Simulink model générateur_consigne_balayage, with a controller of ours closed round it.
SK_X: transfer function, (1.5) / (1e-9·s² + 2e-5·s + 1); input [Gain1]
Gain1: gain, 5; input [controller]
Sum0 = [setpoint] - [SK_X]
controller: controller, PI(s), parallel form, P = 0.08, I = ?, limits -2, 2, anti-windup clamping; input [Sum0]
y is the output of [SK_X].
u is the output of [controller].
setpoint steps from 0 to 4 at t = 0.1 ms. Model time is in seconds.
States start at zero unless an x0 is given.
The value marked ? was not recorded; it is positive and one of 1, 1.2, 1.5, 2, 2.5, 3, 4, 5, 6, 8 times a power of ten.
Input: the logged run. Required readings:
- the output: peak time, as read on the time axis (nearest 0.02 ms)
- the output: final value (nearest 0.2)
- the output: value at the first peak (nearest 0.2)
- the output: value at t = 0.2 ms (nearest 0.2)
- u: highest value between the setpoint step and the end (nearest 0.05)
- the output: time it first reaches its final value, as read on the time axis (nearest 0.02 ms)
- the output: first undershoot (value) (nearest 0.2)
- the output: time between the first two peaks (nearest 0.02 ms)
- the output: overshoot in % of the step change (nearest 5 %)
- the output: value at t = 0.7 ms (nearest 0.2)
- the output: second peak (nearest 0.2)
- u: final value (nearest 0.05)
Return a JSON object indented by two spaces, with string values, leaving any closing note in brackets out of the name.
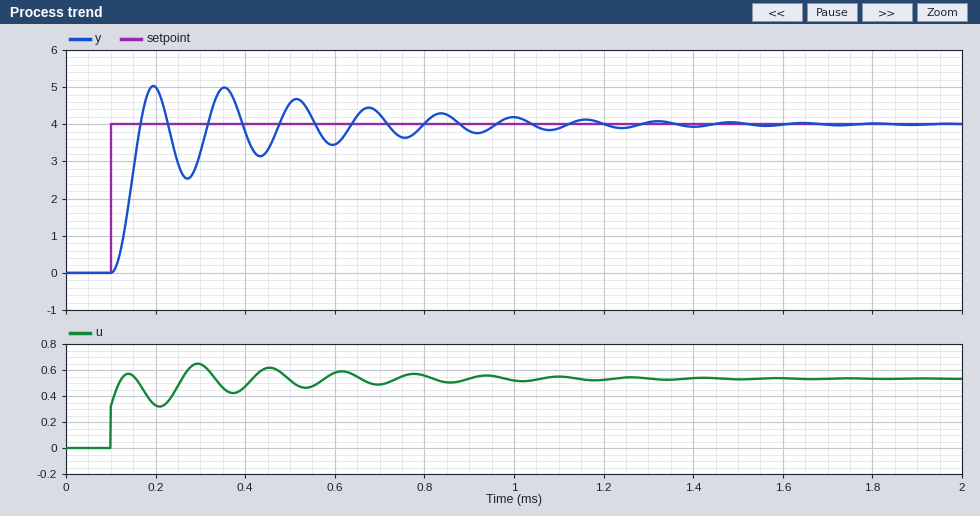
{
  "the output: peak time, as read on the time axis": "0.20 ms",
  "the output: final value": "4.0",
  "the output: value at the first peak": "5.0",
  "the output: value at t = 0.2 ms": "5.0",
  "u: highest value between the setpoint step and the end": "0.65",
  "the output: time it first reaches its final value, as read on the time axis": "0.16 ms",
  "the output: first undershoot (value)": "2.6",
  "the output: time between the first two peaks": "0.16 ms",
  "the output: overshoot in % of the step change": "25 %",
  "the output: value at t = 0.7 ms": "4.2",
  "the output: second peak": "5.0",
  "u: final value": "0.55"
}
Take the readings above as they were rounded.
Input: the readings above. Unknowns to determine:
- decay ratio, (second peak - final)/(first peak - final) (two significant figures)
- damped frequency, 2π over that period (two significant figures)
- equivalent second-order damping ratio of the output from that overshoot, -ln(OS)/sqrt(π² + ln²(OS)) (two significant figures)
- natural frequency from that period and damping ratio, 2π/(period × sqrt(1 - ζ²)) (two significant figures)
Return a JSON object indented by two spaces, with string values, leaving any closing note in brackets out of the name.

{
  "decay ratio, (second peak - final)/(first peak - final)": "1.0",
  "damped frequency, 2π over that period": "39 rad/ms",
  "equivalent second-order damping ratio of the output from that overshoot, -ln(OS)/sqrt(π² + ln²(OS))": "0.40",
  "natural frequency from that period and damping ratio, 2π/(period × sqrt(1 - ζ²))": "43 rad/ms"
}
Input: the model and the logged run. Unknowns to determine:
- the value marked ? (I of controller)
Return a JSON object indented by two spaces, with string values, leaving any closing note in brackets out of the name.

{
  "the value marked ?": "3000"
}
